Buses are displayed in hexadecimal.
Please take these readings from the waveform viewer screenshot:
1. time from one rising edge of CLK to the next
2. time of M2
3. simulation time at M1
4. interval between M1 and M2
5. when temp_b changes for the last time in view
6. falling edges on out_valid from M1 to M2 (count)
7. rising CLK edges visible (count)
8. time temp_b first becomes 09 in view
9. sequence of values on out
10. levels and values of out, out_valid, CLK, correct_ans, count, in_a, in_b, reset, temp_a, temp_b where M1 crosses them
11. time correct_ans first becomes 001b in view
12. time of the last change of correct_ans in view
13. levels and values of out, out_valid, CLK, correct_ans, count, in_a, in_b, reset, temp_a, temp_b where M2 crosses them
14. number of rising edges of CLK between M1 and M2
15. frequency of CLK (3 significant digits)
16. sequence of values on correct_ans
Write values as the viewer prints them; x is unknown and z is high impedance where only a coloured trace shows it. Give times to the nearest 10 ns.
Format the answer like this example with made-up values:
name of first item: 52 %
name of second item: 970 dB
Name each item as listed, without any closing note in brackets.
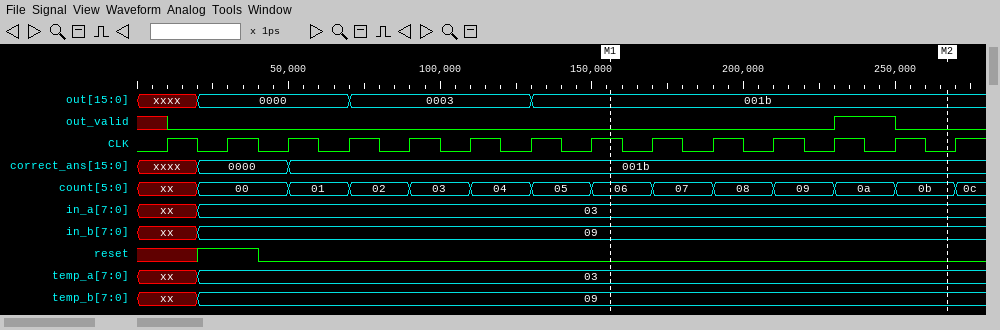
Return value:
time from one rising edge of CLK to the next: 20 ns
time of M2: 270 ns
simulation time at M1: 160 ns
interval between M1 and M2: 110 ns
when temp_b changes for the last time in view: 20 ns
falling edges on out_valid from M1 to M2: 1
rising CLK edges visible: 14
time temp_b first becomes 09 in view: 20 ns
sequence of values on out: xxxx, 0000, 0003, 001b
levels and values of out, out_valid, CLK, correct_ans, count, in_a, in_b, reset, temp_a, temp_b where M1 crosses them: out=001b, out_valid=0, CLK=1, correct_ans=001b, count=06, in_a=03, in_b=09, reset=0, temp_a=03, temp_b=09
time correct_ans first becomes 001b in view: 50 ns
time of the last change of correct_ans in view: 50 ns
levels and values of out, out_valid, CLK, correct_ans, count, in_a, in_b, reset, temp_a, temp_b where M2 crosses them: out=001b, out_valid=0, CLK=0, correct_ans=001b, count=0b, in_a=03, in_b=09, reset=0, temp_a=03, temp_b=09
number of rising edges of CLK between M1 and M2: 5
frequency of CLK: 50.0 MHz
sequence of values on correct_ans: xxxx, 0000, 001b
